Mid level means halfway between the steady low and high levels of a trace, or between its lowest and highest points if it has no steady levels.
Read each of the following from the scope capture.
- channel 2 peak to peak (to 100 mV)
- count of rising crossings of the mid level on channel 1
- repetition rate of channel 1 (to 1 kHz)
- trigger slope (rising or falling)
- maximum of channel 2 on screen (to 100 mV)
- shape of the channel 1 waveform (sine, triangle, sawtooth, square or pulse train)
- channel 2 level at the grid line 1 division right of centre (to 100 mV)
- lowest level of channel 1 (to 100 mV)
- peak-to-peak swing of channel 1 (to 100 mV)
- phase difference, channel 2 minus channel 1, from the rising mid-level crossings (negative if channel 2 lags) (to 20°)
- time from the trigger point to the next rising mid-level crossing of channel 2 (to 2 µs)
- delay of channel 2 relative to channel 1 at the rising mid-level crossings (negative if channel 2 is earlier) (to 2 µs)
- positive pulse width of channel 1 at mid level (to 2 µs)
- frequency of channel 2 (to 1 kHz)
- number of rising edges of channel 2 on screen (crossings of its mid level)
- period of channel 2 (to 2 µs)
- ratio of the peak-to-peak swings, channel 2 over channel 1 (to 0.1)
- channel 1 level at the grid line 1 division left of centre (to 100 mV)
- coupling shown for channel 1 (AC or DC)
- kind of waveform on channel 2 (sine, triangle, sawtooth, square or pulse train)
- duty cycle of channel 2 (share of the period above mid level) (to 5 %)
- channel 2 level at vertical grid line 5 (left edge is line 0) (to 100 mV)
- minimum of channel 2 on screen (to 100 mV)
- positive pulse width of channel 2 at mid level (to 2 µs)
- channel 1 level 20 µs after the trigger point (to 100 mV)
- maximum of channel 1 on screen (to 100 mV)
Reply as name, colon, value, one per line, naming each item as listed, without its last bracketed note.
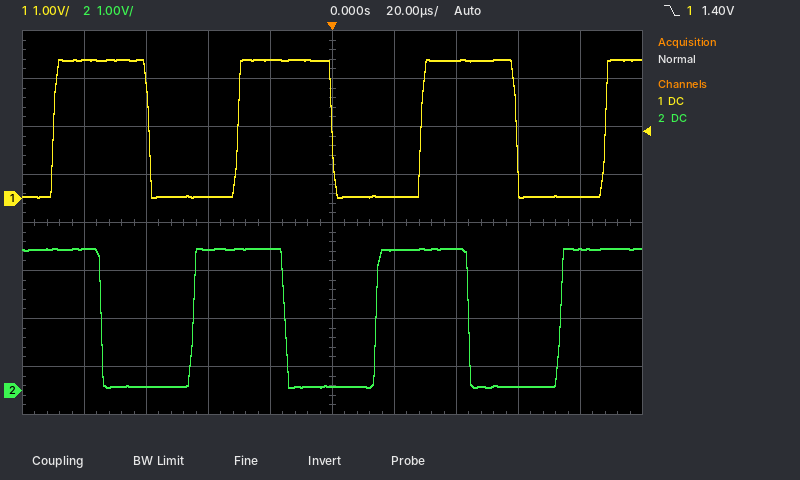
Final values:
channel 2 peak to peak: 2.9 V
count of rising crossings of the mid level on channel 1: 4
repetition rate of channel 1: 17 kHz
trigger slope: falling
maximum of channel 2 on screen: 3.0 V
shape of the channel 1 waveform: square
channel 2 level at the grid line 1 division right of centre: 2.9 V
lowest level of channel 1: 0.0 V
peak-to-peak swing of channel 1: 2.9 V
phase difference, channel 2 minus channel 1, from the rising mid-level crossings (negative if channel 2 lags): +80°
time from the trigger point to the next rising mid-level crossing of channel 2: 14 µs
delay of channel 2 relative to channel 1 at the rising mid-level crossings (negative if channel 2 is earlier): -14 µs
positive pulse width of channel 1 at mid level: 30 µs
frequency of channel 2: 17 kHz
number of rising edges of channel 2 on screen: 3
period of channel 2: 60 µs
ratio of the peak-to-peak swings, channel 2 over channel 1: 1.0
channel 1 level at the grid line 1 division left of centre: 2.9 V
coupling shown for channel 1: DC
kind of waveform on channel 2: square
duty cycle of channel 2 (share of the period above mid level): 50 %
channel 2 level at vertical grid line 5 (left edge is line 0): 100 mV
minimum of channel 2 on screen: 100 mV
positive pulse width of channel 2 at mid level: 30 µs
channel 1 level 20 µs after the trigger point: 0.0 V
maximum of channel 1 on screen: 2.9 V
